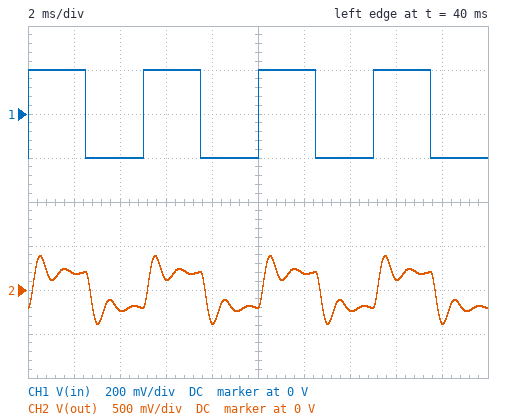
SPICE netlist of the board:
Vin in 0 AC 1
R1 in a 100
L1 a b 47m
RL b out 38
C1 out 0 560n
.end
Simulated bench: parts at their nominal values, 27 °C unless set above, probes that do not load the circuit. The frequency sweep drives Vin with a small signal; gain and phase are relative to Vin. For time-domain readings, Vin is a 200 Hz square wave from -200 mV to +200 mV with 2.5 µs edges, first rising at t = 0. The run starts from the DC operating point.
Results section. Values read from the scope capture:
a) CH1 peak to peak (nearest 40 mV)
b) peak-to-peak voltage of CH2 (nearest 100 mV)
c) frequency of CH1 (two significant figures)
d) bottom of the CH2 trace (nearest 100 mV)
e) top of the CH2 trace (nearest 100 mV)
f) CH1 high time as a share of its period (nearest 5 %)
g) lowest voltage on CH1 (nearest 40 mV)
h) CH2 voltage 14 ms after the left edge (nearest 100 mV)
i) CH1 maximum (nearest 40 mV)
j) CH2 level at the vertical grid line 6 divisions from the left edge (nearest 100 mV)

400 mV
800 mV
200 Hz
-400 mV
400 mV
50 %
-200 mV
-200 mV
200 mV
200 mV
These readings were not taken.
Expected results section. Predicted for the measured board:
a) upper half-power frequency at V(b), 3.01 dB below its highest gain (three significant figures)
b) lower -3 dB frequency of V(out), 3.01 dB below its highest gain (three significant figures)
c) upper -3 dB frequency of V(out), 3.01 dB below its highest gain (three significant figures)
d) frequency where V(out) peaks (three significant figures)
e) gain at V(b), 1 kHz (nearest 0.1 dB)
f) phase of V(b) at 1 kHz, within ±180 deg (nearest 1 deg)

1.14 kHz
639 Hz
1.14 kHz
924 Hz
6.3 dB
-87 deg
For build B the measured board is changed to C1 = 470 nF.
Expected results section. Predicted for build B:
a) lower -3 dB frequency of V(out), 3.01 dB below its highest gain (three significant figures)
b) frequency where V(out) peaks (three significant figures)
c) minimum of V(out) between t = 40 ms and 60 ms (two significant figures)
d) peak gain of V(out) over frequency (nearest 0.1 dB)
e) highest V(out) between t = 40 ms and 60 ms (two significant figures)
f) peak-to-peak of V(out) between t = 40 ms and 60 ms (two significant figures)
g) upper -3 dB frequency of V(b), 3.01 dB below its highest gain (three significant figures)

741 Hz
1.02 kHz
-400 mV
7.4 dB
400 mV
810 mV
1.24 kHz
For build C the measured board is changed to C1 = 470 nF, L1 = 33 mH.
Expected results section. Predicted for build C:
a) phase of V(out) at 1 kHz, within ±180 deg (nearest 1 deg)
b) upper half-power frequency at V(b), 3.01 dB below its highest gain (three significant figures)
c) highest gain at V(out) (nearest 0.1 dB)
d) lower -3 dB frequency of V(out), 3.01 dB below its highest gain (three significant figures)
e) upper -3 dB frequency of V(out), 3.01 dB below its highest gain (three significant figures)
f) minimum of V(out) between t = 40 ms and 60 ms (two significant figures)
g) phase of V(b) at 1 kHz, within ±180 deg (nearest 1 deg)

-46 deg
1.50 kHz
6.0 dB
768 Hz
1.49 kHz
-370 mV
-40 deg
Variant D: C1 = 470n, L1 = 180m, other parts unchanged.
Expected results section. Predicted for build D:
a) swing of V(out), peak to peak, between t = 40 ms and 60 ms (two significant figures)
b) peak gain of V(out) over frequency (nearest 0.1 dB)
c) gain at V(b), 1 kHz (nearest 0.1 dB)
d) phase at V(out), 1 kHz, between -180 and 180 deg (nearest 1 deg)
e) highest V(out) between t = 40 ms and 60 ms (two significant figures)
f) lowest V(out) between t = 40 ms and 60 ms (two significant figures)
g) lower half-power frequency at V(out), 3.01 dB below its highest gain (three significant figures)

1.1 V
13.1 dB
-7.5 dB
-170 deg
530 mV
-530 mV
475 Hz
